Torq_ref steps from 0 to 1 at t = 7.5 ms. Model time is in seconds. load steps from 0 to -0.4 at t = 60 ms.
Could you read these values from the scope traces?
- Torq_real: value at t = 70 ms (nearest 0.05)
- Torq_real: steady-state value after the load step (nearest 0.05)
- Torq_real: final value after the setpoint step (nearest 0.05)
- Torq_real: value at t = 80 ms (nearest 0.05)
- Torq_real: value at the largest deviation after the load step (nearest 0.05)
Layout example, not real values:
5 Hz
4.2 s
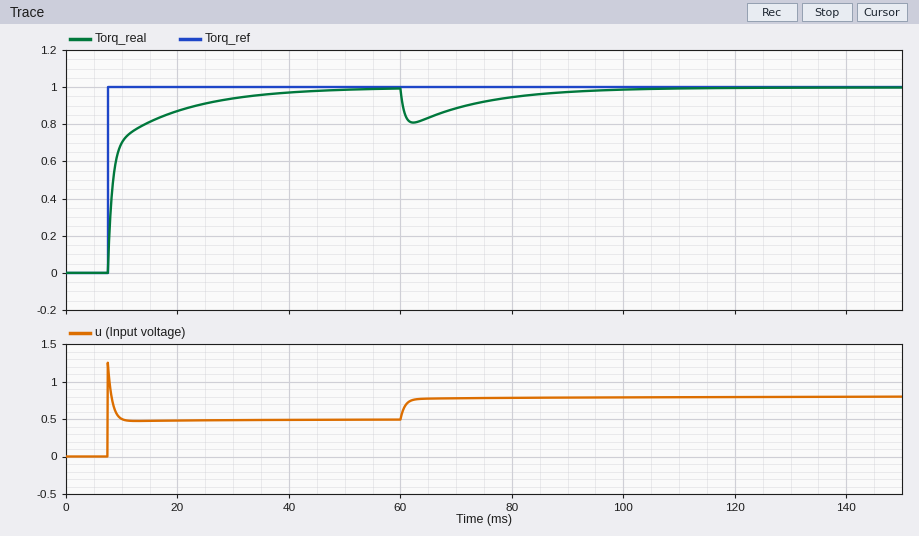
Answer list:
0.90
1.00
1.00
0.95
0.80
